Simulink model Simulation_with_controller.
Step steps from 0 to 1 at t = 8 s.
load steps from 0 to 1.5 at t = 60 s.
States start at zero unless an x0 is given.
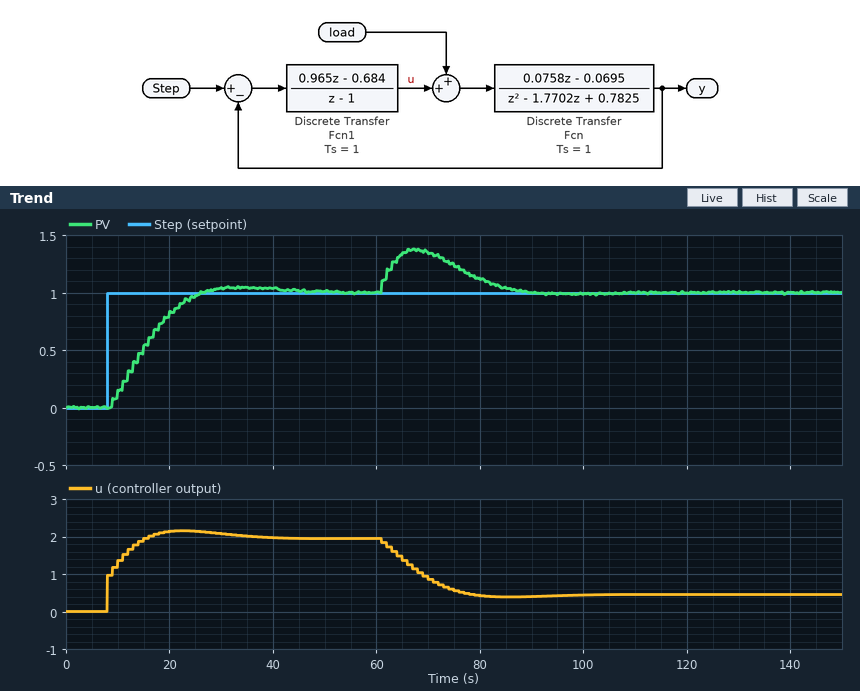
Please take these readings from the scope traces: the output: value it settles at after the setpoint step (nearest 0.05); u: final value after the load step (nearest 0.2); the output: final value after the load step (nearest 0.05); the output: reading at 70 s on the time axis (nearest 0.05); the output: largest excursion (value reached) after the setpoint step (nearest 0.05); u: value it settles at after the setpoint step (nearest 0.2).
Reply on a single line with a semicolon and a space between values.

1.00; 0.4; 1.00; 1.35; 1.05; 2.0
